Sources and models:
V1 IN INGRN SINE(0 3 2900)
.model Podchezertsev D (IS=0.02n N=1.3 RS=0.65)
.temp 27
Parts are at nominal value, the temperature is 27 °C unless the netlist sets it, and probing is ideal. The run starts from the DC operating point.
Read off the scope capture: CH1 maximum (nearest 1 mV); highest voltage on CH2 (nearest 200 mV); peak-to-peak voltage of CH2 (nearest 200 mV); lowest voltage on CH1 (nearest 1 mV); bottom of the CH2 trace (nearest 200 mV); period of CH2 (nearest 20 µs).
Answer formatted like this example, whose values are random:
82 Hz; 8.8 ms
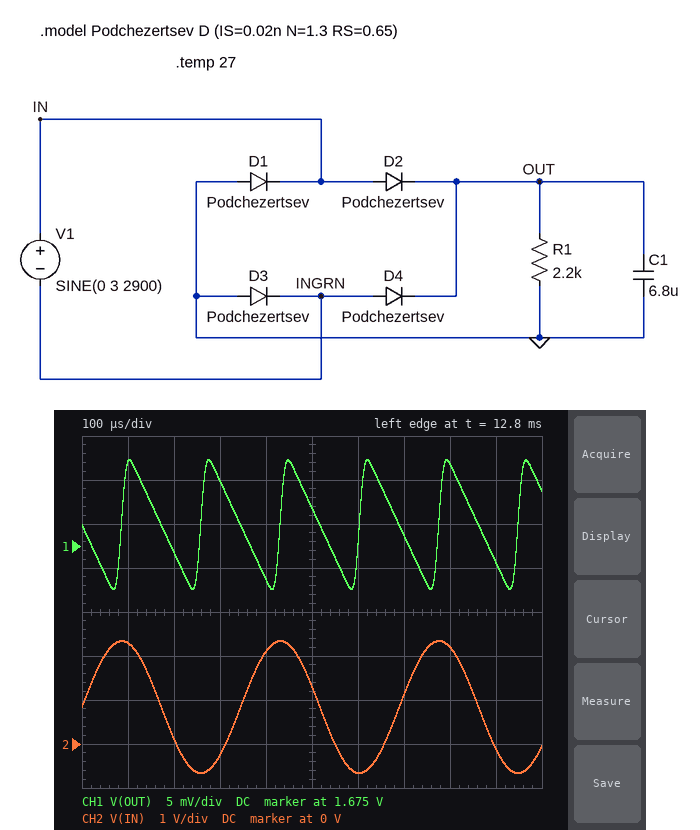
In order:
1.685 V; 2.4 V; 3.0 V; 1.670 V; -600 mV; 340 µs
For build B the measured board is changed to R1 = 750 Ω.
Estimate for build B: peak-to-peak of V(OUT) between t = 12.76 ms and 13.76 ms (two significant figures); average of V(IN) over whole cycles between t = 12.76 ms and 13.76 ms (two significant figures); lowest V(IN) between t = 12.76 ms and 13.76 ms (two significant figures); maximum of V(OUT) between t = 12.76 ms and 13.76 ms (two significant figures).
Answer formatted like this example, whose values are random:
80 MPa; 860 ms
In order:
41 mV; 800 mV; -700 mV; 1.6 V
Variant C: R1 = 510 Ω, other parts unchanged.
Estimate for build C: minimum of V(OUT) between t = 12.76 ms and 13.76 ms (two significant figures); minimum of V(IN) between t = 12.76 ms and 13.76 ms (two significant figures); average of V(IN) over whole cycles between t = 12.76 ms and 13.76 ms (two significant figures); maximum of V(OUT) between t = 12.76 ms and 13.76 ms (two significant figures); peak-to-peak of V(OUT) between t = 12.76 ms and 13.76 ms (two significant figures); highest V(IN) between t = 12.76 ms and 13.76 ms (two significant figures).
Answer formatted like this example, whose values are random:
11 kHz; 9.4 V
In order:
1.5 V; -720 mV; 780 mV; 1.6 V; 58 mV; 2.3 V
